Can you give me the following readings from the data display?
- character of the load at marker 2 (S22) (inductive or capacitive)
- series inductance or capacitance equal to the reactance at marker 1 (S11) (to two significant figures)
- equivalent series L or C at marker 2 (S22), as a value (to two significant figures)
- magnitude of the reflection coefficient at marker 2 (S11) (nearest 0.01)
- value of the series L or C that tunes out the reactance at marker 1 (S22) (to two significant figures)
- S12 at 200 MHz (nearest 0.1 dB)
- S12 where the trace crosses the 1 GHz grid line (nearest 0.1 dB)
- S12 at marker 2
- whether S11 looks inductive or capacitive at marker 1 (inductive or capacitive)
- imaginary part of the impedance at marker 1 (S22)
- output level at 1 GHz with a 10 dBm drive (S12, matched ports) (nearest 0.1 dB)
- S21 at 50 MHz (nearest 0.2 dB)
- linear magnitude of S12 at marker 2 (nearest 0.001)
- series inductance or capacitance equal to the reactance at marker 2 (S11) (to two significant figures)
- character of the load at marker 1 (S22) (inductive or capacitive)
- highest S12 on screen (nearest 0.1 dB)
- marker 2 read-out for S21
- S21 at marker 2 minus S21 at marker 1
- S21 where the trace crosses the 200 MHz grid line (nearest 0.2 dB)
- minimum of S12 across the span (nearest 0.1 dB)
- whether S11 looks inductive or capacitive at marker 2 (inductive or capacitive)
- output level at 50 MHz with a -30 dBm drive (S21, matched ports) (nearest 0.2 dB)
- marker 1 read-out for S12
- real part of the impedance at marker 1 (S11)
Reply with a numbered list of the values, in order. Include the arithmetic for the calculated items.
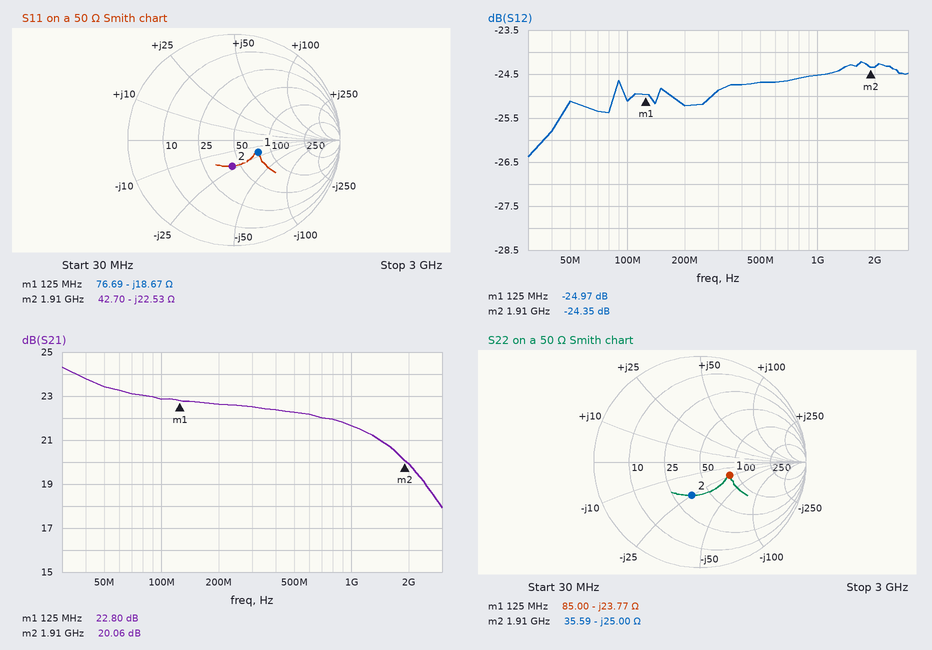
1. capacitive
2. C = 1/(2π × 125 MHz × 18.67 Ω) ≈ 68 pF
3. C = 1/(2π × 1.91 GHz × 25 Ω) ≈ 3.3 pF
4. 0.25
5. L = 23.77 Ω/(2π × 125 MHz) ≈ 30 nH
6. -25.2 dB
7. -24.5 dB
8. -24.35 dB
9. capacitive
10. -23.77 Ω
11. 10 dBm + (-24.5 dB) = -14.5 dBm
12. 23.4 dB
13. 10^(-24.35/20) ≈ 0.061
14. C = 1/(2π × 1.91 GHz × 22.53 Ω) ≈ 3.7 pF
15. capacitive
16. -24.2 dB
17. 20.06 dB
18. 20.06 − (22.8) = -2.74 dB
19. 22.6 dB
20. -26.4 dB
21. capacitive
22. -30 dBm + (23.4 dB) = -6.6 dBm
23. -24.97 dB
24. 76.69 Ω
